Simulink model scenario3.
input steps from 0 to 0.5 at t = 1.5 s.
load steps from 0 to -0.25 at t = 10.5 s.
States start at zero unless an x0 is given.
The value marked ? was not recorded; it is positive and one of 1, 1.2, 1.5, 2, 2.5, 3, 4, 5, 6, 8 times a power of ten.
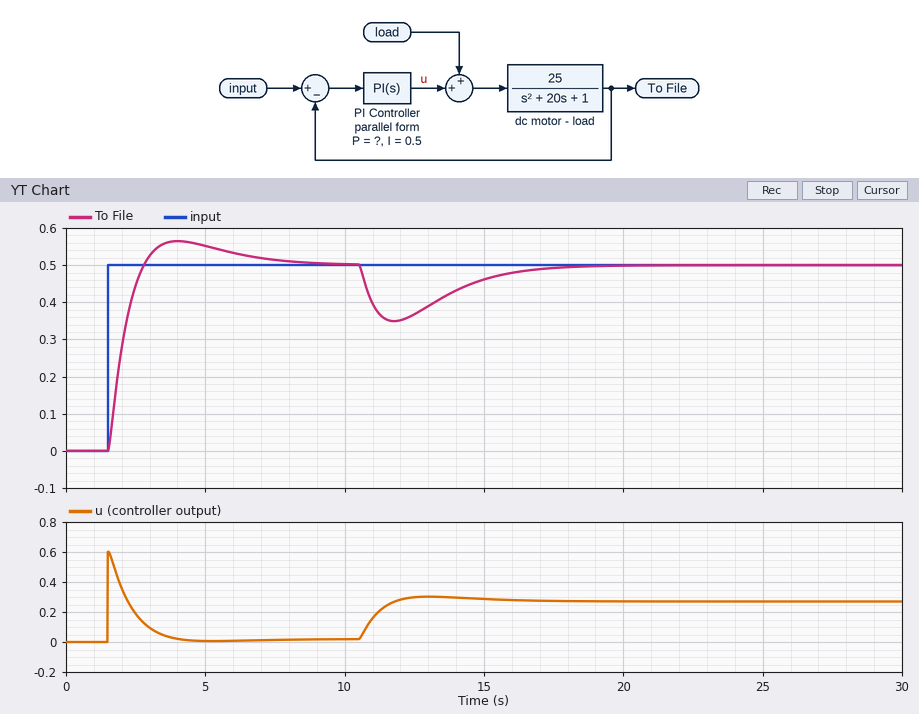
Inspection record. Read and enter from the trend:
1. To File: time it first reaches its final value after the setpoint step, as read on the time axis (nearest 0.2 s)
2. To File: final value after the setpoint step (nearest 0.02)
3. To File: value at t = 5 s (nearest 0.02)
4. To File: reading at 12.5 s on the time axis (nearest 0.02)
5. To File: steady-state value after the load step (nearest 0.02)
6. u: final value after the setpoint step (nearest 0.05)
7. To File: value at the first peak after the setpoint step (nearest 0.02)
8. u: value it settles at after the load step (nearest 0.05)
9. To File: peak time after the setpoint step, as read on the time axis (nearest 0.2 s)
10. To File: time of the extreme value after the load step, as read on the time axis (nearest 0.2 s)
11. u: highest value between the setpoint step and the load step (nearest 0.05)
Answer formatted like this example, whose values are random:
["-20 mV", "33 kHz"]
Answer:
["2.8 s", "0.50", "0.56", "0.36", "0.50", "0.00", "0.56", "0.25", "4.0 s", "11.8 s", "0.60"]
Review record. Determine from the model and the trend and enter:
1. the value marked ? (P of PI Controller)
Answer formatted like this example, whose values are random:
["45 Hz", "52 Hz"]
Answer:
["1.2"]
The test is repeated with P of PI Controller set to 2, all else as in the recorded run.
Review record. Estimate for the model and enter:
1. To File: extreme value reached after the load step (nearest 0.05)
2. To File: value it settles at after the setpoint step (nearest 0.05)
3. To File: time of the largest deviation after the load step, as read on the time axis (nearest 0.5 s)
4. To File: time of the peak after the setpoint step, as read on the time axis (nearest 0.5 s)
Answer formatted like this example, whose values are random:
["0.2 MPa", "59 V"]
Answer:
["0.40", "0.50", "11.5 s", "3.5 s"]
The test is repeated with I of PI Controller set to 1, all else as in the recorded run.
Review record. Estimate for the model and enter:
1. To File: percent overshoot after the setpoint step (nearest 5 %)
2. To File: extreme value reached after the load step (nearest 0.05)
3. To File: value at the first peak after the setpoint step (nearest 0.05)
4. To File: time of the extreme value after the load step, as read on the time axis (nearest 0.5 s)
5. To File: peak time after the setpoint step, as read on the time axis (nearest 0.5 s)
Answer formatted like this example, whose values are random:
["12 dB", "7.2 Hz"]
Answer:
["20 %", "0.35", "0.60", "11.5 s", "3.5 s"]
